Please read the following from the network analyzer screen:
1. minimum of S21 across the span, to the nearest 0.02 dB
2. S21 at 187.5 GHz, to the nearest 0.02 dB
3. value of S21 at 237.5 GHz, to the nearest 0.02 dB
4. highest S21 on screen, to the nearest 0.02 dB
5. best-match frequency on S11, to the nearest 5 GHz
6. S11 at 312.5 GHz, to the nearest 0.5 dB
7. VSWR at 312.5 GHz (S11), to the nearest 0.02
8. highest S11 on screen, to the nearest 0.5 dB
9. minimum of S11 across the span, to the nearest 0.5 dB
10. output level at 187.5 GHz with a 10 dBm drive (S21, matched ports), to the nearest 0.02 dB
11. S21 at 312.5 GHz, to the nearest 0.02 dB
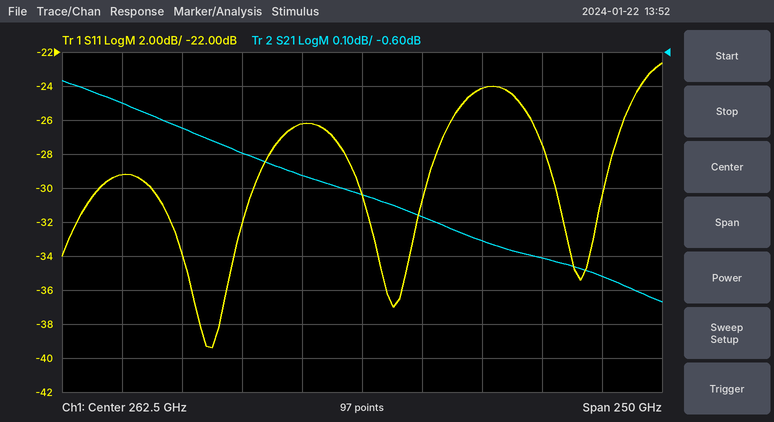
-1.34 dB
-0.82 dB
-0.96 dB
-0.68 dB
200 GHz
-24.0 dB
1.14
-22.5 dB
-39.5 dB
9.18 dBm
-1.16 dB
